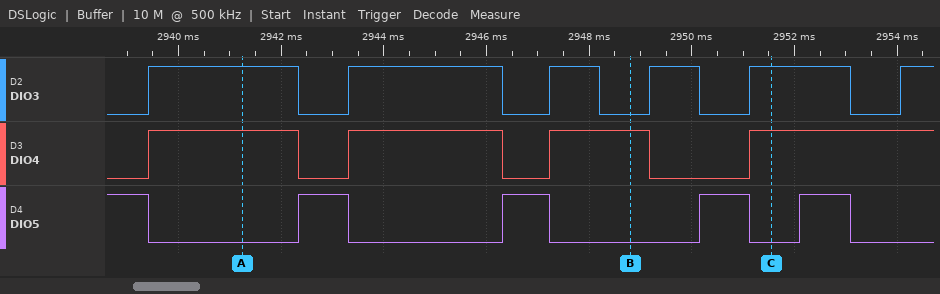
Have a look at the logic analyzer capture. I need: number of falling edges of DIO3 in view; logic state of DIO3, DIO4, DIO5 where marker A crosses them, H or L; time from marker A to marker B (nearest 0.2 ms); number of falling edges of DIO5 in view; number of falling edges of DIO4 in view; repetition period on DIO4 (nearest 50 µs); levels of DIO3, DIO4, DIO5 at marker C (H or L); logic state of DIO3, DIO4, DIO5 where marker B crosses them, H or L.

5
DIO3=H, DIO4=H, DIO5=L
7.6 ms
5
3
3900 µs
DIO3=H, DIO4=H, DIO5=L
DIO3=L, DIO4=H, DIO5=L
